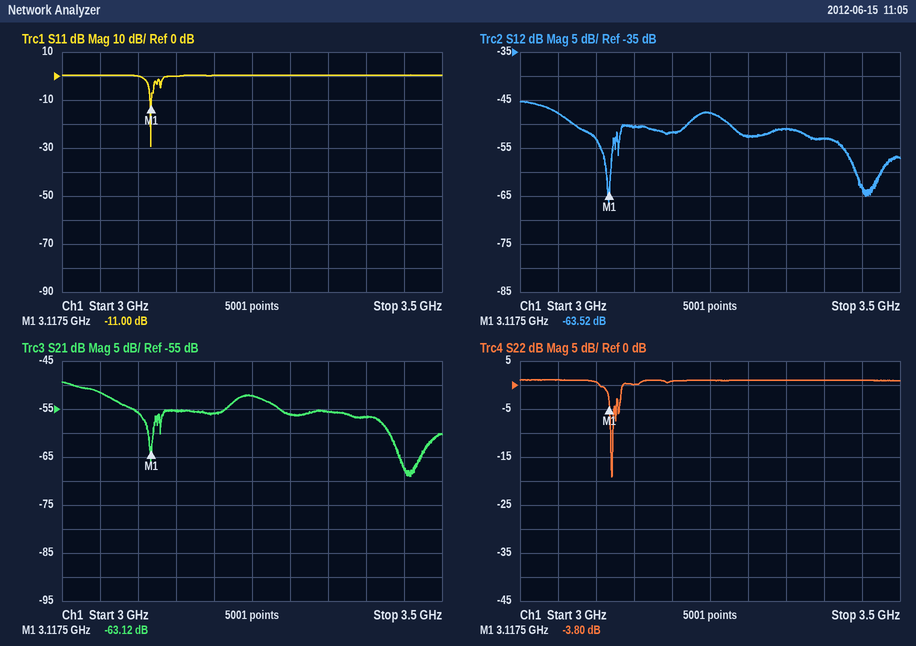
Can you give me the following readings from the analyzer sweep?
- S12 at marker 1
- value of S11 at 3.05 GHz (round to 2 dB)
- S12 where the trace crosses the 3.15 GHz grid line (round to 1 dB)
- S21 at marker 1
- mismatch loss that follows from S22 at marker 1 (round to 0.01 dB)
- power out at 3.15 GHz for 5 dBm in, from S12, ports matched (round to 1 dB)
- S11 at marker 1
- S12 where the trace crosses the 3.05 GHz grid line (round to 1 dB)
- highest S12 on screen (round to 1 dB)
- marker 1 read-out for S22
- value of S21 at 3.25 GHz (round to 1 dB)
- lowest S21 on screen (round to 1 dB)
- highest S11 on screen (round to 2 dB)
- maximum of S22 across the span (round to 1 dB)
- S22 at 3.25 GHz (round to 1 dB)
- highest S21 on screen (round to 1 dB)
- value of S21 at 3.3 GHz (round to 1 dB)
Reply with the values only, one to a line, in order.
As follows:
-63.52 dB
0 dB
-51 dB
-63.12 dB
2.34 dB
-46 dBm
-11.00 dB
-48 dB
-45 dB
-3.80 dB
-52 dB
-69 dB
0 dB
1 dB
1 dB
-49 dB
-56 dB
